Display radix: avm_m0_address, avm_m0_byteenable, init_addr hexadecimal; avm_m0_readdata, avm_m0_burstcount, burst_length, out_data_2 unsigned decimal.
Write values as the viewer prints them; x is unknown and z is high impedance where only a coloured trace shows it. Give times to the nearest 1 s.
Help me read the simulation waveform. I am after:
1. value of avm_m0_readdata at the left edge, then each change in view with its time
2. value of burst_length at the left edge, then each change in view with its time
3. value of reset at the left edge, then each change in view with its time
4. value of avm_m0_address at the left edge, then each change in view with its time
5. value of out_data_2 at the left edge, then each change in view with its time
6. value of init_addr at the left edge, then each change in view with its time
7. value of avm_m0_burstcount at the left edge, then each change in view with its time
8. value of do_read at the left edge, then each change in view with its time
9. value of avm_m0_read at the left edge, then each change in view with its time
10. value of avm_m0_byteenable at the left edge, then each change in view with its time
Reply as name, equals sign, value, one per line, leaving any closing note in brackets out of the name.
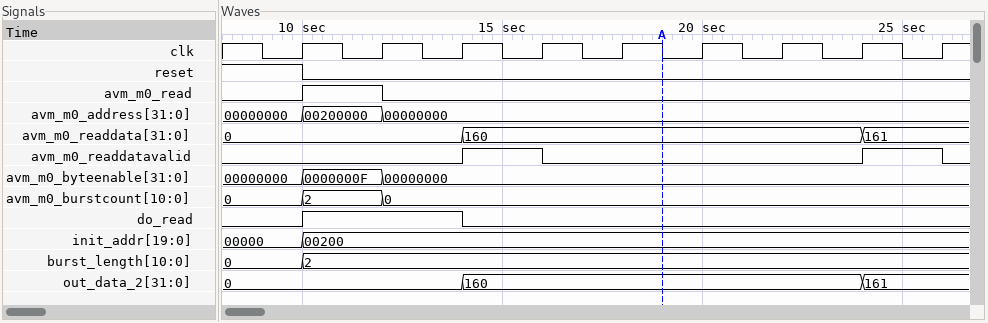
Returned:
value of avm_m0_readdata at the left edge, then each change in view with its time = 0, 160 at 14 s, 161 at 24 s
value of burst_length at the left edge, then each change in view with its time = 0, 2 at 10 s
value of reset at the left edge, then each change in view with its time = 1, 0 at 10 s
value of avm_m0_address at the left edge, then each change in view with its time = 00000000, 00200000 at 10 s, 00000000 at 12 s
value of out_data_2 at the left edge, then each change in view with its time = 0, 160 at 14 s, 161 at 24 s
value of init_addr at the left edge, then each change in view with its time = 00000, 00200 at 10 s
value of avm_m0_burstcount at the left edge, then each change in view with its time = 0, 2 at 10 s, 0 at 12 s
value of do_read at the left edge, then each change in view with its time = 0, 1 at 10 s, 0 at 14 s
value of avm_m0_read at the left edge, then each change in view with its time = 0, 1 at 10 s, 0 at 12 s
value of avm_m0_byteenable at the left edge, then each change in view with its time = 00000000, 0000000F at 10 s, 00000000 at 12 s
